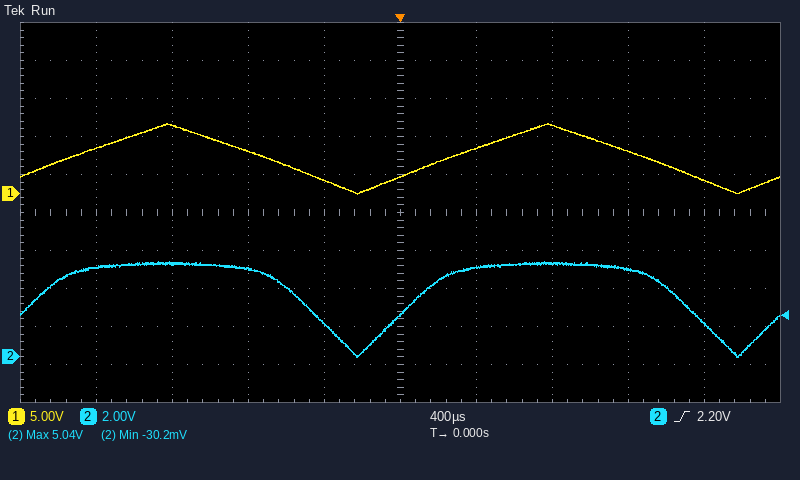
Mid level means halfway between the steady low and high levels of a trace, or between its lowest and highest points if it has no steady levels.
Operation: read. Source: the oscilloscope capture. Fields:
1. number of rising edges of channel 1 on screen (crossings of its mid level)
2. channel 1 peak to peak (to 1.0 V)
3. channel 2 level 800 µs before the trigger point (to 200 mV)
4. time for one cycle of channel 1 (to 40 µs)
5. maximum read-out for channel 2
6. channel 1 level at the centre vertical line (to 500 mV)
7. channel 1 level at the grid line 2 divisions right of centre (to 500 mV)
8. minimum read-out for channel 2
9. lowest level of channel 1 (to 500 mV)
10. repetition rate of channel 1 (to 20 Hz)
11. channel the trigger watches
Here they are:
2
9.0 V
4.6 V
2.00 ms
5.04 V
2.0 V
9.0 V
-30.2 mV
0.0 V
500 Hz
channel 2
